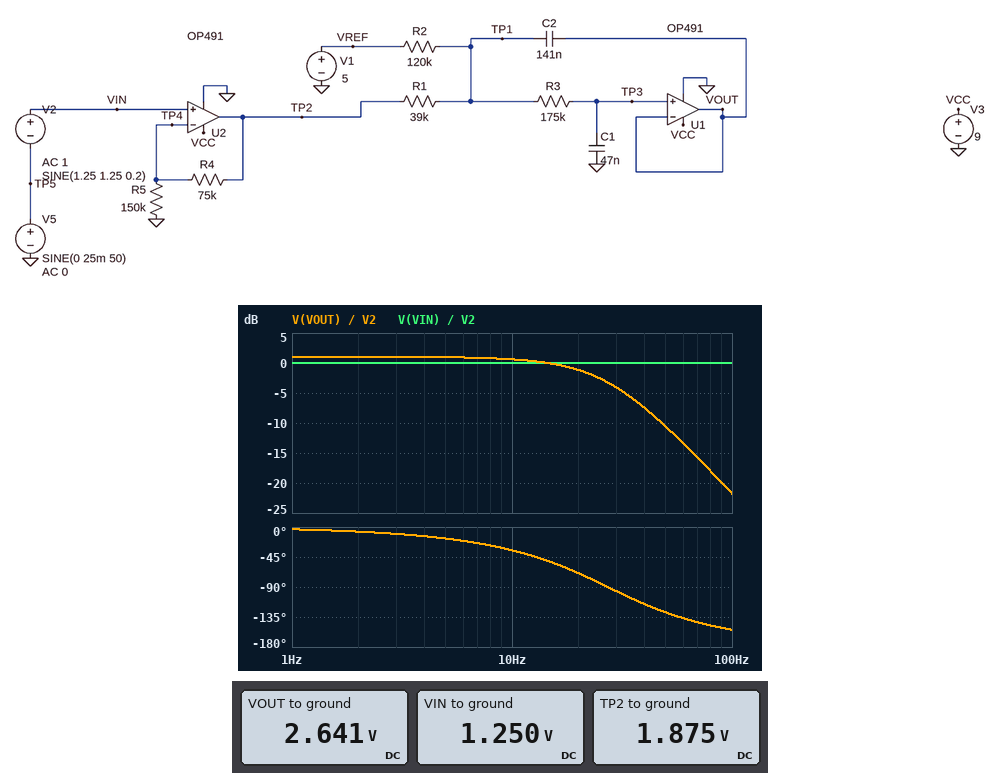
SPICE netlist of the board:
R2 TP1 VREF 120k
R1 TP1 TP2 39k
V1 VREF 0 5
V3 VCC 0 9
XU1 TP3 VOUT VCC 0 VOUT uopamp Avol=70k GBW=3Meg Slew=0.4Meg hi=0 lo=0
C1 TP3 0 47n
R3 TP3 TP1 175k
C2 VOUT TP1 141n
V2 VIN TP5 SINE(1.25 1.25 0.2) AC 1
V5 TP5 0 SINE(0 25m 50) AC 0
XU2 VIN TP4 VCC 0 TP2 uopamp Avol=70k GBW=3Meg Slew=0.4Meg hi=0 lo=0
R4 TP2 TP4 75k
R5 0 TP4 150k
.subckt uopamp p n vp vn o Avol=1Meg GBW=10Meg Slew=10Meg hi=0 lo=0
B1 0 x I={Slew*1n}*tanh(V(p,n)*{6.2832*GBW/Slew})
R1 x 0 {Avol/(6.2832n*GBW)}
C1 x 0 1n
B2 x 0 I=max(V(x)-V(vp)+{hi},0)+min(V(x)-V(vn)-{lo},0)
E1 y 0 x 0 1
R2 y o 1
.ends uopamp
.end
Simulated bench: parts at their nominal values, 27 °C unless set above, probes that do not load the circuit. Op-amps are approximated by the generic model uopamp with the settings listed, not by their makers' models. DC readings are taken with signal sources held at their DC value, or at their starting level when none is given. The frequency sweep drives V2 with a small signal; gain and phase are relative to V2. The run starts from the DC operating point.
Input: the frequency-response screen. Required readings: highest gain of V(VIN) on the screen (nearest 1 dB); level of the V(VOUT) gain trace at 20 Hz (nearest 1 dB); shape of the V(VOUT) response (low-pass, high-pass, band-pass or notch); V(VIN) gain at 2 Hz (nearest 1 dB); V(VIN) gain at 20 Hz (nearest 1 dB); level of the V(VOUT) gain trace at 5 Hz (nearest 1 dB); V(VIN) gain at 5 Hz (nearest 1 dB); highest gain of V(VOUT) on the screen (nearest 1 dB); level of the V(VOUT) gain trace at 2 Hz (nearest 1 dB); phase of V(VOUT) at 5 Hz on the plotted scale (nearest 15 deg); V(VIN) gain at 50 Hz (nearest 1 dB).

0 dB
-1 dB
low-pass
0 dB
0 dB
1 dB
0 dB
1 dB
1 dB
-15 deg
0 dB
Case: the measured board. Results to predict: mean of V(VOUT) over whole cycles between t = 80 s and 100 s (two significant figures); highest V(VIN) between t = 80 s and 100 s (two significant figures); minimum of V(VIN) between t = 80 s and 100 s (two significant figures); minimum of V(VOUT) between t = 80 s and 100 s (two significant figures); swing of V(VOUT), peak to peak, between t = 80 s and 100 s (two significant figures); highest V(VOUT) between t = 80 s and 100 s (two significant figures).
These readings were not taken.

2.6 V
2.5 V
-25 mV
1.2 V
2.8 V
4.1 V
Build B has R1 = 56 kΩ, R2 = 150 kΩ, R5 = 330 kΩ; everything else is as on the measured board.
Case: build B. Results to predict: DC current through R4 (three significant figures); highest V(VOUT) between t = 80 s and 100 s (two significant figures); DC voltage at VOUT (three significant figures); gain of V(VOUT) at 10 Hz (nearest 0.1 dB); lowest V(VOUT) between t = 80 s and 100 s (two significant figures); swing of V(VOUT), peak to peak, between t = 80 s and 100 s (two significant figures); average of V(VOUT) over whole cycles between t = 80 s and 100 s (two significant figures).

3.79 µA
3.6 V
2.48 V
-1.3 dB
1.4 V
2.2 V
2.5 V
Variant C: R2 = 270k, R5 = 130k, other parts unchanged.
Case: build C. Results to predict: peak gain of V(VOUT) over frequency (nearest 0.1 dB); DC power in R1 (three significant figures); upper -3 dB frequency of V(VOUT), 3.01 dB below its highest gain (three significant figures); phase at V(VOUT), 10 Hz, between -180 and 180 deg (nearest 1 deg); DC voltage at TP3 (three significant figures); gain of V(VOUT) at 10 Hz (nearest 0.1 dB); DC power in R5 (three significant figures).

2.8 dB
3.75 µW
22.7 Hz
-36 deg
2.35 V
2.4 dB
12.0 µW
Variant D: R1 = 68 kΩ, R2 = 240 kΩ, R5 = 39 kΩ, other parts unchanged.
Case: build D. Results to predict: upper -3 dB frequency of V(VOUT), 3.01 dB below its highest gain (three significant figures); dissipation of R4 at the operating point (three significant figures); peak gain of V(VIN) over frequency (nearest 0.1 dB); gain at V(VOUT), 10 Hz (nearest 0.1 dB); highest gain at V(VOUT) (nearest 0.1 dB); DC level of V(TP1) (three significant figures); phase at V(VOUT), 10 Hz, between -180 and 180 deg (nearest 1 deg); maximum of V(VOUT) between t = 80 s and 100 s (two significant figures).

20.9 Hz
77.0 µW
0 dB
7.0 dB
7.2 dB
3.95 V
-42 deg
6.8 V
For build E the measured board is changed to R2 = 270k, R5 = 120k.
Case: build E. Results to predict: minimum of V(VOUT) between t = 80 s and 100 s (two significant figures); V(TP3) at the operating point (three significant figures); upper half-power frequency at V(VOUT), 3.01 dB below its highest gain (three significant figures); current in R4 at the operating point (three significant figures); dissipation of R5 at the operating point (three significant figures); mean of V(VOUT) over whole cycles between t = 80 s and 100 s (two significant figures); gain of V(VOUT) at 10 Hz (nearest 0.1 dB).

640 mV
2.41 V
22.7 Hz
10.4 µA
13.0 µW
2.4 V
2.7 dB
